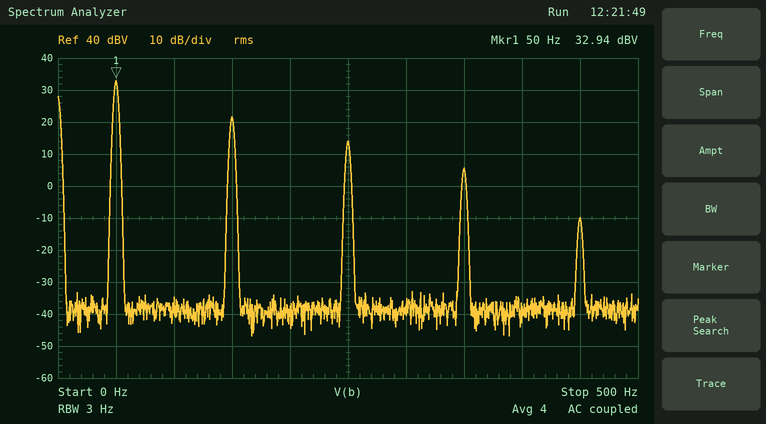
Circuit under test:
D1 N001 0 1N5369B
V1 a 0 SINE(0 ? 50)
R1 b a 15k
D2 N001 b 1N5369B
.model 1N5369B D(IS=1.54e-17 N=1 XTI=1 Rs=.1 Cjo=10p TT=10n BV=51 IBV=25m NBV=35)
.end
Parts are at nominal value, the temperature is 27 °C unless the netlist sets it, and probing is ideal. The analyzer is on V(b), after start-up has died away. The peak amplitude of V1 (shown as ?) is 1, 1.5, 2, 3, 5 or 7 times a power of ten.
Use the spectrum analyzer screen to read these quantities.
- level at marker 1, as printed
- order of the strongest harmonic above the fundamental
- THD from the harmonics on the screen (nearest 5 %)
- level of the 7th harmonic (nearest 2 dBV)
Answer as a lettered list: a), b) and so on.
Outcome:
a) 32.94 dBV
b) 3
c) 30 %
d) 6 dBV
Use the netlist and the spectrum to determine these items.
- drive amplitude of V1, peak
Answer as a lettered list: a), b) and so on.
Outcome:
a) 150 V
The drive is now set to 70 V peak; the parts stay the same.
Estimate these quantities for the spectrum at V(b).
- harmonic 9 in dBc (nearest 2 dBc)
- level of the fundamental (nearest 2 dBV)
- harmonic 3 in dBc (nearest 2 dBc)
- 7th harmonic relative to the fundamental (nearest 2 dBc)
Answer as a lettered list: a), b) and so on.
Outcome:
a) -50 dBc
b) 32 dBV
c) -18 dBc
d) -34 dBc
